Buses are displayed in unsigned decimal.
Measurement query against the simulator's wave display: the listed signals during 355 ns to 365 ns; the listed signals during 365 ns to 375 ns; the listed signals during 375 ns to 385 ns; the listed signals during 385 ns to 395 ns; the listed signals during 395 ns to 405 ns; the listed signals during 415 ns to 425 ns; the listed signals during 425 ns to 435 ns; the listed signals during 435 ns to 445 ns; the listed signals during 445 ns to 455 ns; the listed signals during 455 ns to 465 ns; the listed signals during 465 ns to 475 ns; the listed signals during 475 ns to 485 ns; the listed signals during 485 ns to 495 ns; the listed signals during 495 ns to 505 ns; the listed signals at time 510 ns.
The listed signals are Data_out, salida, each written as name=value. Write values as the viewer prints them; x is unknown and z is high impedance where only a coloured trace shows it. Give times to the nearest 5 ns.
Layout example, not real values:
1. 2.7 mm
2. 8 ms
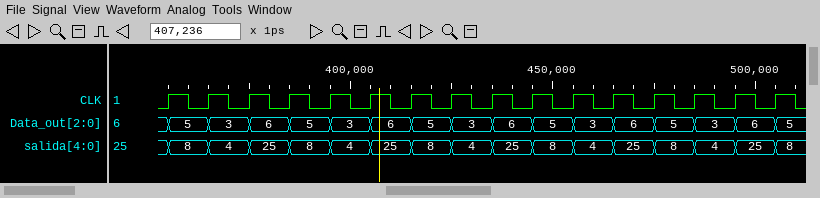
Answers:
1. Data_out=5, salida=8
2. Data_out=3, salida=4
3. Data_out=6, salida=25
4. Data_out=5, salida=8
5. Data_out=3, salida=4
6. Data_out=5, salida=8
7. Data_out=3, salida=4
8. Data_out=6, salida=25
9. Data_out=5, salida=8
10. Data_out=3, salida=4
11. Data_out=6, salida=25
12. Data_out=5, salida=8
13. Data_out=3, salida=4
14. Data_out=6, salida=25
15. Data_out=5, salida=8
